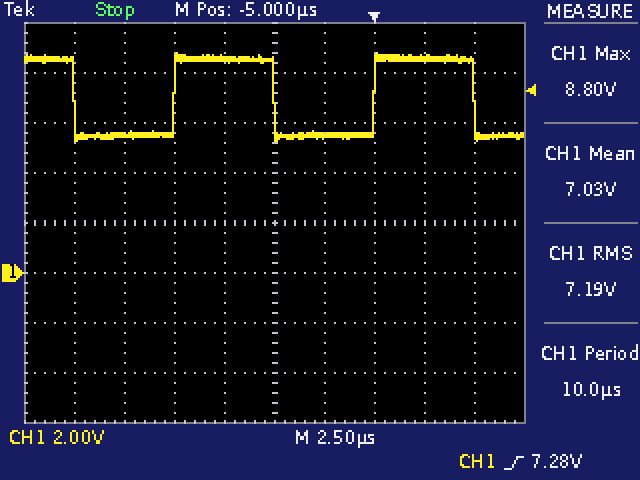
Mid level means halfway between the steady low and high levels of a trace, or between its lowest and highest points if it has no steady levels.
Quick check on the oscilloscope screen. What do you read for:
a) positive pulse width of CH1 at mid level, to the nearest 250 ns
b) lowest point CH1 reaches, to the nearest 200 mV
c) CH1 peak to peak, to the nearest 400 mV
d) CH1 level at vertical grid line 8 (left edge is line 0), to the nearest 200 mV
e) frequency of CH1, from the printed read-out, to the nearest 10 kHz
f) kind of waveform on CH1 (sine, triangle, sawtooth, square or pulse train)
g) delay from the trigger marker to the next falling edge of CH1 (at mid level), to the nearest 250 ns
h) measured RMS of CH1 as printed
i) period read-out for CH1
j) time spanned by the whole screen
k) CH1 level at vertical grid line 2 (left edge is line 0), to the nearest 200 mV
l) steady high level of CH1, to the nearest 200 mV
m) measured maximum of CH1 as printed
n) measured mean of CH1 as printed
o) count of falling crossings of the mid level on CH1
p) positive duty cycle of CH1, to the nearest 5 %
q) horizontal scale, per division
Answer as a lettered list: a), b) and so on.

a) 5.00 µs
b) 5.2 V
c) 3.6 V
d) 8.6 V
e) 100 kHz
f) square
g) 5.00 µs
h) 7.19 V
i) 10.0 µs
j) 25 µs
k) 5.6 V
l) 8.6 V
m) 8.80 V
n) 7.03 V
o) 3
p) 50 %
q) 2.5 µs
